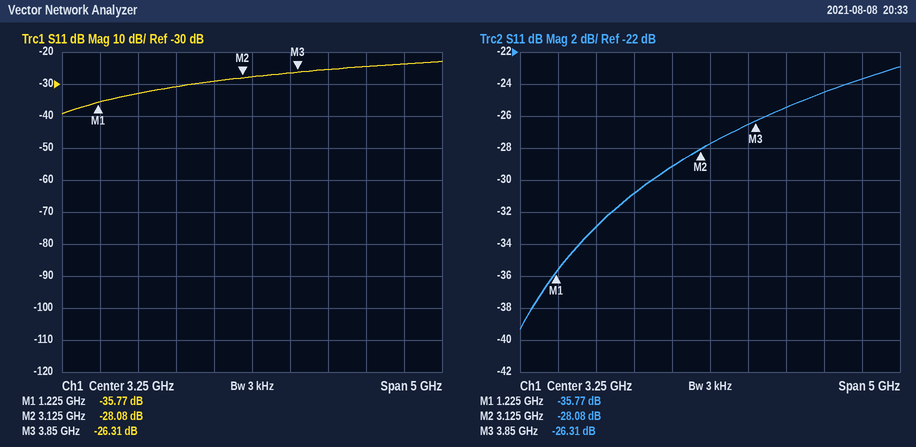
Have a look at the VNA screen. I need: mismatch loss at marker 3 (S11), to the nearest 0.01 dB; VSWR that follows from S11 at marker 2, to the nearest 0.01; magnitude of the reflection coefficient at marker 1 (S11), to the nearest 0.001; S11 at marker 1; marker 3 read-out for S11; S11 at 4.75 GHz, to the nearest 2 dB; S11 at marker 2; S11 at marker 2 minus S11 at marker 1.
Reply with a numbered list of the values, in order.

1. 0.01 dB
2. 1.08
3. 0.016
4. -35.77 dB
5. -26.31 dB
6. -24 dB
7. -28.08 dB
8. 7.69 dB
